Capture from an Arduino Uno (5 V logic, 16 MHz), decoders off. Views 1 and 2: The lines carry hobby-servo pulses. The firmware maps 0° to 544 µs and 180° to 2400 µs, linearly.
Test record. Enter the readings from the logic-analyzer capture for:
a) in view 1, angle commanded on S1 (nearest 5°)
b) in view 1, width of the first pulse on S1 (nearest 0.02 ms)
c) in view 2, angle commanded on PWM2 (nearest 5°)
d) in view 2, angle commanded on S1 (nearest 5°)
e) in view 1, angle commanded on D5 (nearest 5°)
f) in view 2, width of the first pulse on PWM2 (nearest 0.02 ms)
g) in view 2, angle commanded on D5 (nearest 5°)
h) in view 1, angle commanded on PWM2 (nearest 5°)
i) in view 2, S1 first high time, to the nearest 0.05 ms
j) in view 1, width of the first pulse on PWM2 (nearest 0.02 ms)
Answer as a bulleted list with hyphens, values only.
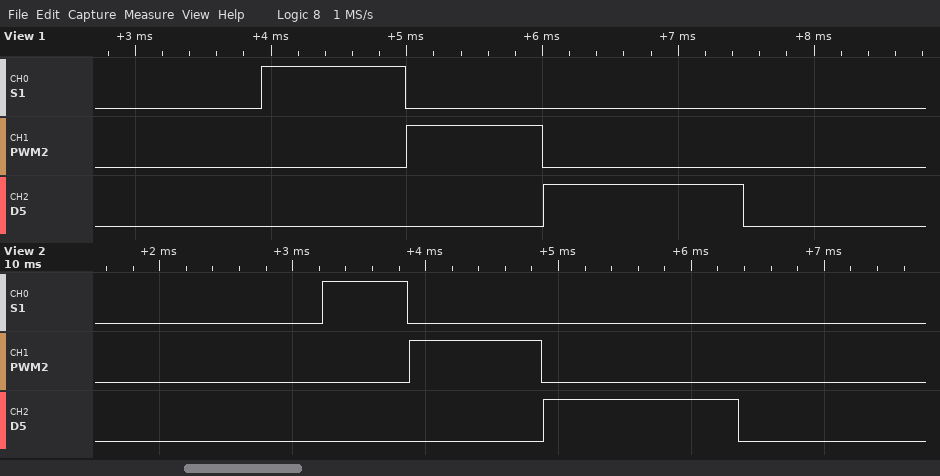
- 50°
- 1.06 ms
- 45°
- 10°
- 90°
- 1.00 ms
- 90°
- 45°
- 0.65 ms
- 1.00 ms
